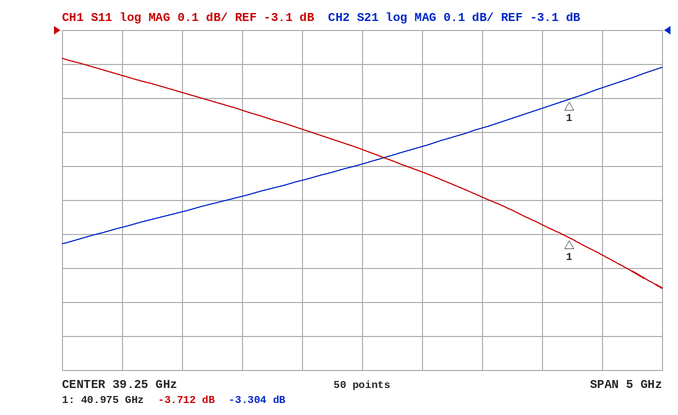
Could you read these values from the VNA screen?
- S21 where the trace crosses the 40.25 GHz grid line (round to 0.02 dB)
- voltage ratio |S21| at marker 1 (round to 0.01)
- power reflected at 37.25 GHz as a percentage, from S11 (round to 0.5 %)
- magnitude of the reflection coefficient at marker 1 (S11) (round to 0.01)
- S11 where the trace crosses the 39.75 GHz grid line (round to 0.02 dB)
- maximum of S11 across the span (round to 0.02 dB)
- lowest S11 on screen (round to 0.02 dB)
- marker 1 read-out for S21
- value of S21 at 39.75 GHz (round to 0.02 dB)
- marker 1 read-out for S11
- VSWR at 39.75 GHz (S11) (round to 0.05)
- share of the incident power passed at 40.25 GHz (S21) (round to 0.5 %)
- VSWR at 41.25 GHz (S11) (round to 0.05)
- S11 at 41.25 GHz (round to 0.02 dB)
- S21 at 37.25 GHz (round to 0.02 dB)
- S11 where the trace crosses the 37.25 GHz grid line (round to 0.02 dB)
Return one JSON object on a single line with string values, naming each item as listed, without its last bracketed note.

{"S21 where the trace crosses the 40.25 GHz grid line": "-3.38 dB", "voltage ratio |S21| at marker 1": "0.68", "power reflected at 37.25 GHz as a percentage, from S11": "47.5 %", "magnitude of the reflection coefficient at marker 1 (S11)": "0.65", "S11 where the trace crosses the 39.75 GHz grid line": "-3.52 dB", "maximum of S11 across the span": "-3.18 dB", "lowest S11 on screen": "-3.86 dB", "marker 1 read-out for S21": "-3.304 dB", "value of S21 at 39.75 GHz": "-3.44 dB", "marker 1 read-out for S11": "-3.712 dB", "VSWR at 39.75 GHz (S11)": "5.00", "share of the incident power passed at 40.25 GHz (S21)": "46.0 %", "VSWR at 41.25 GHz (S11)": "4.70", "S11 at 41.25 GHz": "-3.76 dB", "S21 at 37.25 GHz": "-3.68 dB", "S11 where the trace crosses the 37.25 GHz grid line": "-3.24 dB"}
